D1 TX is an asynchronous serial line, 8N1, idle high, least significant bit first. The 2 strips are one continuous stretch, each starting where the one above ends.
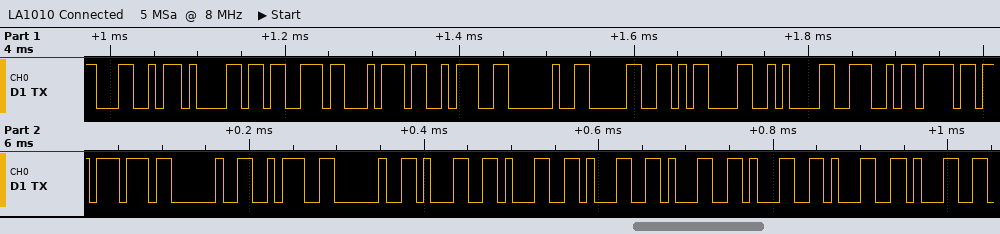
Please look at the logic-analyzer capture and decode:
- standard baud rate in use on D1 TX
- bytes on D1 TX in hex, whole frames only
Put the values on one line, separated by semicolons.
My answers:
115200 baud; 4C 61 73 74 3A 20 30 0D 0A 4E 6F 77 20 3A 20 31 31 31 31 31 31 31
